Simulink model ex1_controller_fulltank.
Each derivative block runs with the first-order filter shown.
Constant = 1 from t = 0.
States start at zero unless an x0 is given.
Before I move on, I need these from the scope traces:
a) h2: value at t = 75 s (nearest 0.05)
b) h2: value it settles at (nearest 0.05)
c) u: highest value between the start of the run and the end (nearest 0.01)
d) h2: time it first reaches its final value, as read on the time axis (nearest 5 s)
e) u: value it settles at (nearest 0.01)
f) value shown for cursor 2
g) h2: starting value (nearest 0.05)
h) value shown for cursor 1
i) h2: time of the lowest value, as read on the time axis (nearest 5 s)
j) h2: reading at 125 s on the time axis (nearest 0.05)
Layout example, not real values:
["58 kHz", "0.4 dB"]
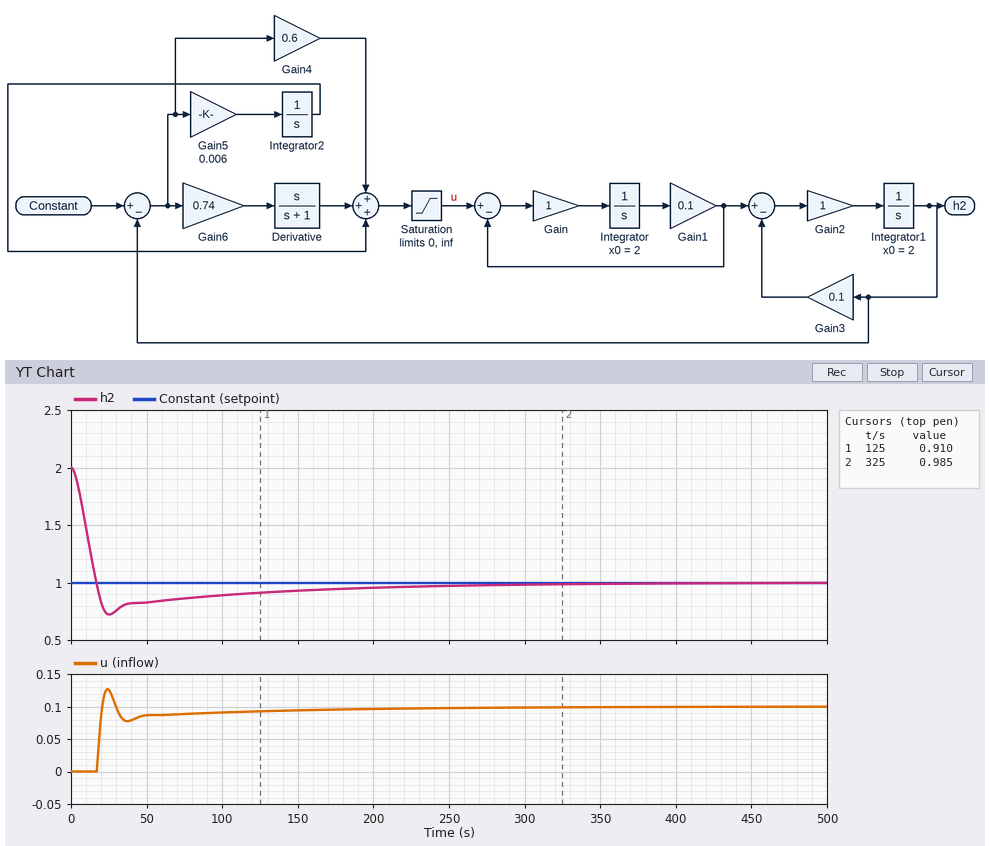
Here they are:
["0.85", "1.00", "0.13", "15 s", "0.10", "0.985", "2.00", "0.910", "25 s", "0.90"]
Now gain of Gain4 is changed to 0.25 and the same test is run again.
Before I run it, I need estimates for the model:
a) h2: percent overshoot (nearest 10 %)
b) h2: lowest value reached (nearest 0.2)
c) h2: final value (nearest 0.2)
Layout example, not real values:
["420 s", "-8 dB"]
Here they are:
["40 %", "0.6", "1.0"]
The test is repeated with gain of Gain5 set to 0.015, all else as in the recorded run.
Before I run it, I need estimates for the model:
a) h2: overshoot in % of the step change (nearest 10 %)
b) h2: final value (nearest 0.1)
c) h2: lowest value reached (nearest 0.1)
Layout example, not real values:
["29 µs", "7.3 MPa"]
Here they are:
["40 %", "1.0", "0.6"]
